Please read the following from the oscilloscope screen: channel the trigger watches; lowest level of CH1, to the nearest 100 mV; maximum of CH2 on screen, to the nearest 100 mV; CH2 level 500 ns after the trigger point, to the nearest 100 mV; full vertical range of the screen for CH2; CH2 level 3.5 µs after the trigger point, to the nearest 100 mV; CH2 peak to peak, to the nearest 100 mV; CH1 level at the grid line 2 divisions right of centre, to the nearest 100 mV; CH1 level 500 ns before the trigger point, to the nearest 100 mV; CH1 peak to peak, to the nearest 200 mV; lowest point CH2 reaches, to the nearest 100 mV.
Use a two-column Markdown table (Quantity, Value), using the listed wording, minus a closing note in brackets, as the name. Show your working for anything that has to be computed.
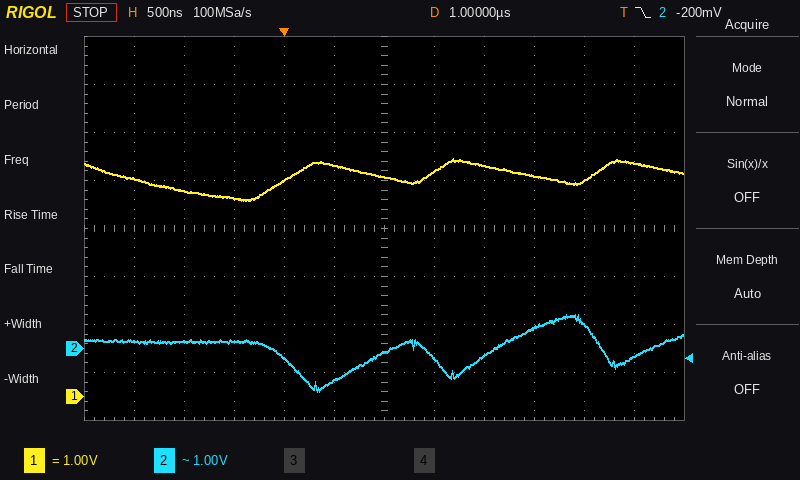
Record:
| Quantity | Value |
|---|---|
| channel the trigger watches | CH2 |
| lowest level of CH1, to the nearest 100 mV | 4.1 V |
| maximum of CH2 on screen, to the nearest 100 mV | 700 mV |
| CH2 level 500 ns after the trigger point, to the nearest 100 mV | -700 mV |
| full vertical range of the screen for CH2 | 8 V |
| CH2 level 3.5 µs after the trigger point, to the nearest 100 mV | -200 mV |
| CH2 peak to peak, to the nearest 100 mV | 700 mV − (-900 mV) = 1.6 V |
| CH1 level at the grid line 2 divisions right of centre, to the nearest 100 mV | 4.8 V |
| CH1 level 500 ns before the trigger point, to the nearest 100 mV | 4.1 V |
| CH1 peak to peak, to the nearest 200 mV | 800 mV |
| lowest point CH2 reaches, to the nearest 100 mV | -900 mV |
